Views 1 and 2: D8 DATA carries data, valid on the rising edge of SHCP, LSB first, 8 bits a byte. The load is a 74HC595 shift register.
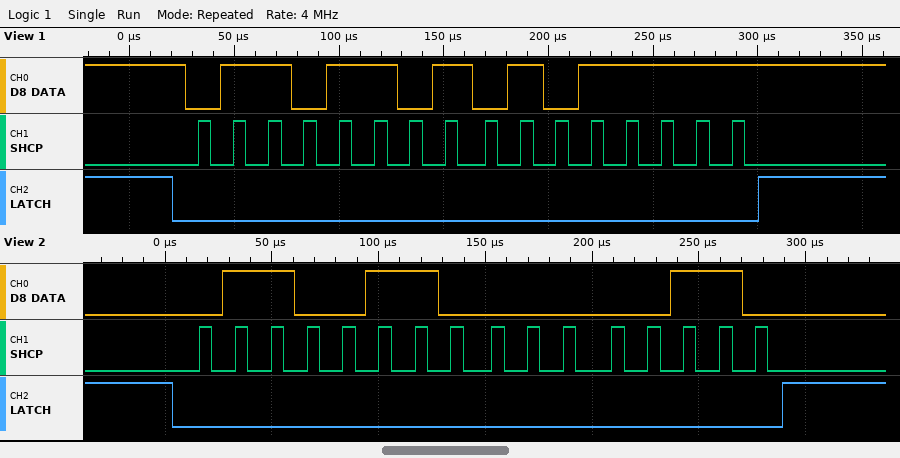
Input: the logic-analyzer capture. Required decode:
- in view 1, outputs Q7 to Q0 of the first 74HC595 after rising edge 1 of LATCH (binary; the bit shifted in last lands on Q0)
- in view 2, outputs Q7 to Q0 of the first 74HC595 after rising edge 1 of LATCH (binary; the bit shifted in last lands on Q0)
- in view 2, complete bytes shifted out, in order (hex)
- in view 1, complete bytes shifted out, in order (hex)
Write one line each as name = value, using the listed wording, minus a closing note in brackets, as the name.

in view 1, outputs Q7 to Q0 of the first 74HC595 after rising edge 1 of LATCH = 01011111
in view 2, outputs Q7 to Q0 of the first 74HC595 after rising edge 1 of LATCH = 00000110
in view 2, complete bytes shifted out, in order = 0x66 0x60
in view 1, complete bytes shifted out, in order = B6 FA
